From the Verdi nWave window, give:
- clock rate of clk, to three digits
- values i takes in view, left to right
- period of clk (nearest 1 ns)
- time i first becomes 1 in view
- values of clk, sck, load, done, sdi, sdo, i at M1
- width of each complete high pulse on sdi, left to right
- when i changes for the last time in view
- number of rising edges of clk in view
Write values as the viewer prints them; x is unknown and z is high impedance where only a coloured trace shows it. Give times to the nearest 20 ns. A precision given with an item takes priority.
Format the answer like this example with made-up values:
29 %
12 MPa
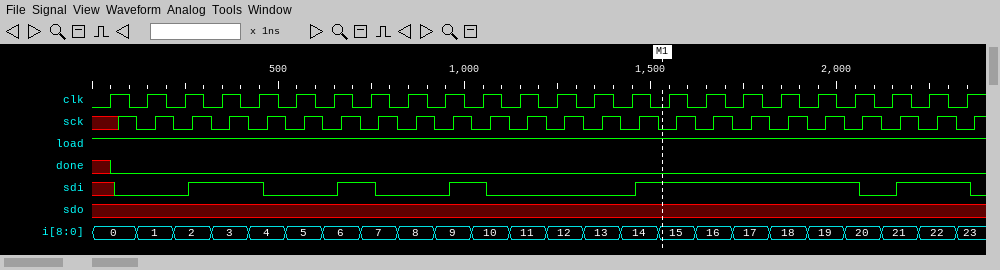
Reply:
10.0 MHz
0, 1, 2, 3, 4, 5, 6, 7, 8, 9, 10, 11, 12, 13, 14, 15, 16, 17, 18, 19, 20, 21, 22, 23
100 ns
120 ns
clk=0, sck=0, load=1, done=0, sdi=1, sdo=x, i=15
200 ns, 100 ns, 100 ns, 600 ns, 200 ns
2320 ns
24
